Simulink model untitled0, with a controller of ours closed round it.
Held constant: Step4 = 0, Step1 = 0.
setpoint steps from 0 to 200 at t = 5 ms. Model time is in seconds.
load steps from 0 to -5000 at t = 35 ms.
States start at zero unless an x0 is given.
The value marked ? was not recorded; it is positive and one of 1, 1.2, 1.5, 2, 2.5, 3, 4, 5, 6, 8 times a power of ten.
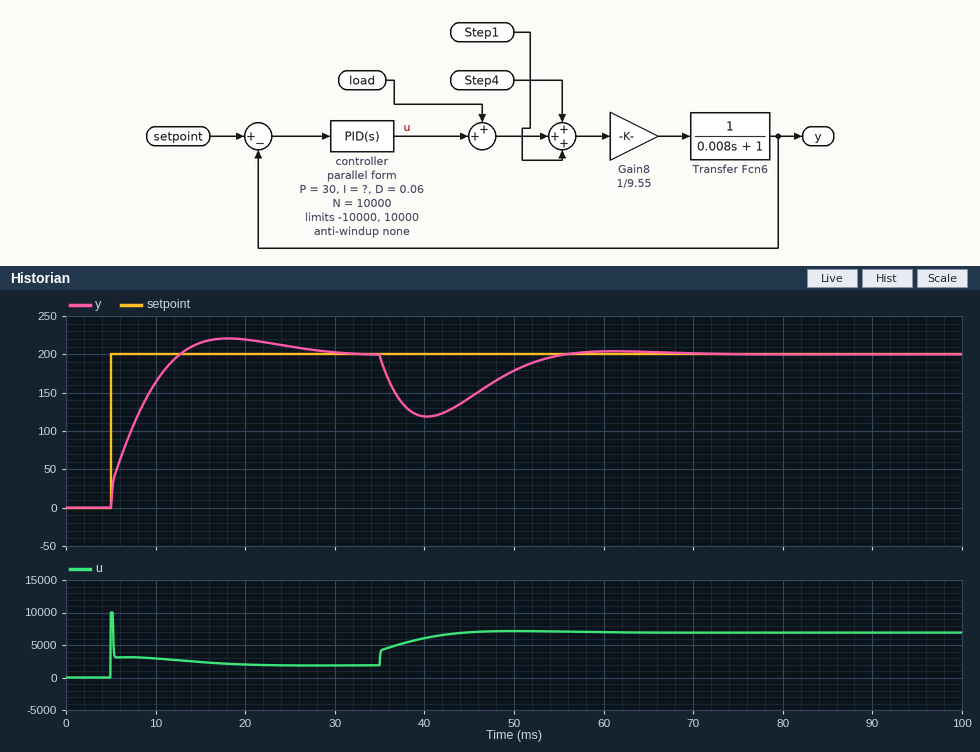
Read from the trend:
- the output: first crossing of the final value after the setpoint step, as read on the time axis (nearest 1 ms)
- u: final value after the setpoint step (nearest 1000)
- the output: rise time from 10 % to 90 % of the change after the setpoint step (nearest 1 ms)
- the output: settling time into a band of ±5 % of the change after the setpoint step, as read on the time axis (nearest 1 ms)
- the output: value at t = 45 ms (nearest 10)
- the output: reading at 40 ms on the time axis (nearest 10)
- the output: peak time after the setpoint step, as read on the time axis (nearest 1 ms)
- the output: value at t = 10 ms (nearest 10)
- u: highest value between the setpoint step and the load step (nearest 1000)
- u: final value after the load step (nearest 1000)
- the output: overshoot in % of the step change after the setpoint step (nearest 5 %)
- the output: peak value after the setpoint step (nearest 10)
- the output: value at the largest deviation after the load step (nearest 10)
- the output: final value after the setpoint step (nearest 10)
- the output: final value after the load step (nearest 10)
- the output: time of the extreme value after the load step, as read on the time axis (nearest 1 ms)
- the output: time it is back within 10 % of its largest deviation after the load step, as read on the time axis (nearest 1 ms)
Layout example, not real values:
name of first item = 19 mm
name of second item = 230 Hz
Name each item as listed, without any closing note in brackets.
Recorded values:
the output: first crossing of the final value after the setpoint step, as read on the time axis = 13 ms
u: final value after the setpoint step = 2000
the output: rise time from 10 % to 90 % of the change after the setpoint step = 6 ms
the output: settling time into a band of ±5 % of the change after the setpoint step, as read on the time axis = 25 ms
the output: value at t = 45 ms = 140
the output: reading at 40 ms on the time axis = 120
the output: peak time after the setpoint step, as read on the time axis = 18 ms
the output: value at t = 10 ms = 160
u: highest value between the setpoint step and the load step = 10000
u: final value after the load step = 7000
the output: overshoot in % of the step change after the setpoint step = 10 %
the output: peak value after the setpoint step = 220
the output: value at the largest deviation after the load step = 120
the output: final value after the setpoint step = 200
the output: final value after the load step = 200
the output: time of the extreme value after the load step, as read on the time axis = 40 ms
the output: time it is back within 10 % of its largest deviation after the load step, as read on the time axis = 53 ms
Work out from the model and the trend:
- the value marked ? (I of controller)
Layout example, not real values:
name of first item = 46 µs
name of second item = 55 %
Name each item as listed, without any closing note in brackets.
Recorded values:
the value marked ? = 6000
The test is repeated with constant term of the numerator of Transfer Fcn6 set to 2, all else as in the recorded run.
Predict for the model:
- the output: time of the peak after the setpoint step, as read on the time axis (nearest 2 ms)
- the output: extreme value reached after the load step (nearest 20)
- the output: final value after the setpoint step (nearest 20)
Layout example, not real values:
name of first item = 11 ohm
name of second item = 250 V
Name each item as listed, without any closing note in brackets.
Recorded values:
the output: time of the peak after the setpoint step, as read on the time axis = 16 ms
the output: extreme value reached after the load step = 100
the output: final value after the setpoint step = 200
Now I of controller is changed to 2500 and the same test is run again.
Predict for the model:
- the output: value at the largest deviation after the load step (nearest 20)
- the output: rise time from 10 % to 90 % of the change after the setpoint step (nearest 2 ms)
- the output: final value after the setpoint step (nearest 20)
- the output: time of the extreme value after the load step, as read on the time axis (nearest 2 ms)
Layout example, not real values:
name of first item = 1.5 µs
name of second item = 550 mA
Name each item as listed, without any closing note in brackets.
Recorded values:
the output: value at the largest deviation after the load step = 100
the output: rise time from 10 % to 90 % of the change after the setpoint step = 10 ms
the output: final value after the setpoint step = 200
the output: time of the extreme value after the load step, as read on the time axis = 42 ms
